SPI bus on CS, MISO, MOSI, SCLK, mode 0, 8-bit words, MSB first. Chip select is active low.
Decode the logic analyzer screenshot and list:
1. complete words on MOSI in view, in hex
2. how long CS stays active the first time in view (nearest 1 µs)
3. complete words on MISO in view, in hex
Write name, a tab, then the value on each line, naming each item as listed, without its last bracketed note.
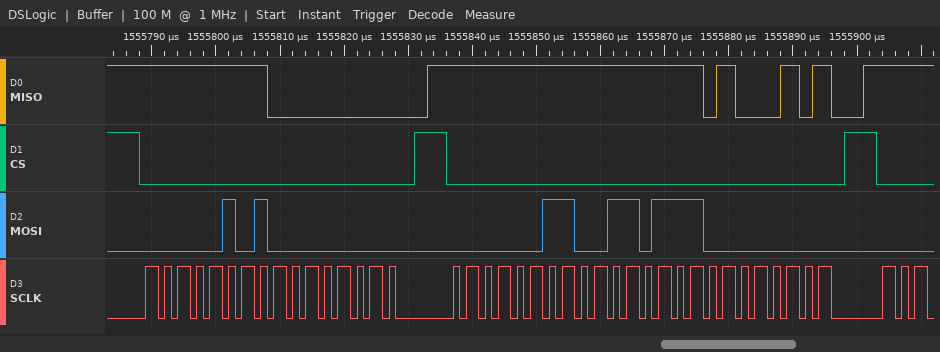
complete words on MOSI in view, in hex	05, 00, 03, 37, 00
how long CS stays active the first time in view	43 µs
complete words on MISO in view, in hex	FF, 00, FF, FF, 45
